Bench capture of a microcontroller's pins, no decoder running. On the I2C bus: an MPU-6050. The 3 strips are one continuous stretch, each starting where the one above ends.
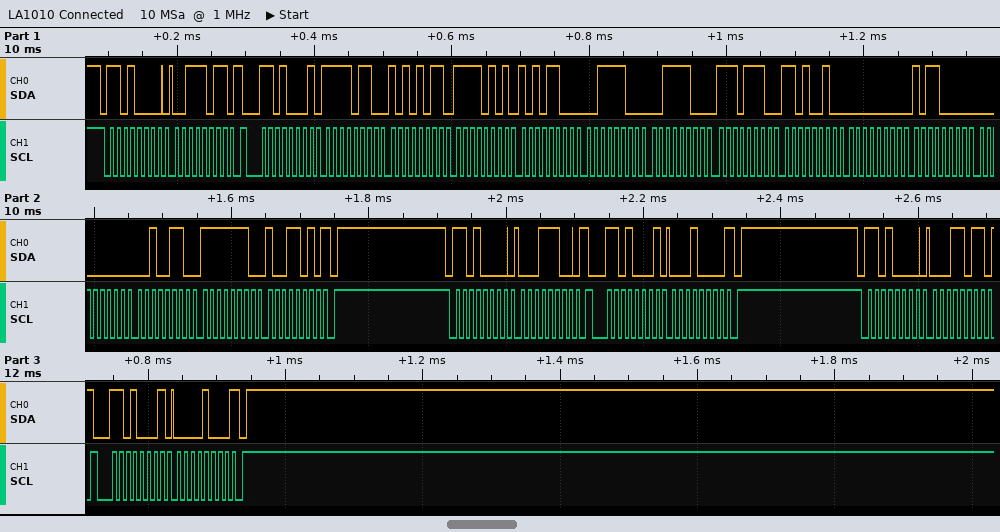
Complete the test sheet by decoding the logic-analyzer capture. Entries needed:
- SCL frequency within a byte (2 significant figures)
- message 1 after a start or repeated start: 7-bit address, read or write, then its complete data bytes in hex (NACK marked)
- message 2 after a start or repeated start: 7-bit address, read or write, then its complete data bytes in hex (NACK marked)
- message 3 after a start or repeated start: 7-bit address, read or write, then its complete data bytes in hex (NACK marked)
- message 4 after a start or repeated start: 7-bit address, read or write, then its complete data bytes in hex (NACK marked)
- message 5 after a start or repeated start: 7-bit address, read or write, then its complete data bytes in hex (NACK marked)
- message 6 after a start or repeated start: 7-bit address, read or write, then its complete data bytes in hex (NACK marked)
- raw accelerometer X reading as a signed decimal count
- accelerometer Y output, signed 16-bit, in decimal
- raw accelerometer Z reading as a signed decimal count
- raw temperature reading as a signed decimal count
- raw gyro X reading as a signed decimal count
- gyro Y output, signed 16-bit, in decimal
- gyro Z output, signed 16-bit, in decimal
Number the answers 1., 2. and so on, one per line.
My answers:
1. 100 kHz
2. 0x68 write: 3B
3. 0x68 read: F6 AB F5 AC 3C 3C EE D2 00 B0 00 26 FE 9A NACK
4. 0x68 write: 1C
5. 0x68 read: 10 NACK
6. 0x68 write: 1B
7. 0x68 read: 08 NACK
8. -2389
9. -2644
10. 15420
11. -4398
12. 176
13. 38
14. -358
